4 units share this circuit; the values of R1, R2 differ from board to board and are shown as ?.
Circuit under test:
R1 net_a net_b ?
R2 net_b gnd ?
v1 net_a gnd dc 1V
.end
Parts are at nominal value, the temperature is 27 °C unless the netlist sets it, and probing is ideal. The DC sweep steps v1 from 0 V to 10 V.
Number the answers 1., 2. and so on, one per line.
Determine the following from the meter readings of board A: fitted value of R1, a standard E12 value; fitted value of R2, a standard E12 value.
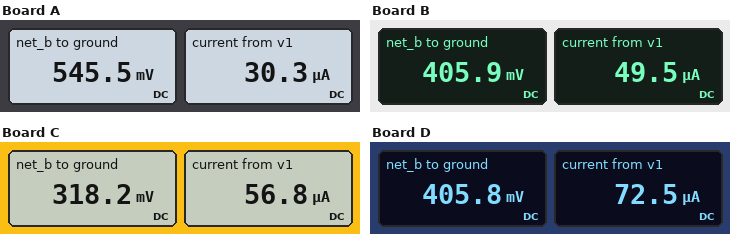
1. 15 kΩ
2. 18 kΩ
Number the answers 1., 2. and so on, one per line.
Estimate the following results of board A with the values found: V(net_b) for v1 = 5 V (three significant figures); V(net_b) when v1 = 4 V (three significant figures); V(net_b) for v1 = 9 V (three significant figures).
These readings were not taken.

1. 2.73 V
2. 2.18 V
3. 4.91 V
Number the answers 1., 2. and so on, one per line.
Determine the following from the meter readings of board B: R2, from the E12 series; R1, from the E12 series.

1. 8.2 kΩ
2. 12 kΩ
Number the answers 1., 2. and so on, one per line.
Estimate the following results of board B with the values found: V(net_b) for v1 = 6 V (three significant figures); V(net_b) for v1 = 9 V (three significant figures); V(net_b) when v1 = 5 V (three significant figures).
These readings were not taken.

1. 2.44 V
2. 3.65 V
3. 2.03 V
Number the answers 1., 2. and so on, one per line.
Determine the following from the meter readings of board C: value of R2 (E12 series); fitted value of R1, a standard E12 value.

1. 5.6 kΩ
2. 12 kΩ
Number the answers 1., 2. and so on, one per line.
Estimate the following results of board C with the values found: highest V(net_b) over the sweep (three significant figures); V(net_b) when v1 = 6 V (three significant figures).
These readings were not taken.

1. 3.18 V
2. 1.91 V
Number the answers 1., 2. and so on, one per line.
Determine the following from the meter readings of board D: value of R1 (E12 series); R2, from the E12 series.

1. 8.2 kΩ
2. 5.6 kΩ
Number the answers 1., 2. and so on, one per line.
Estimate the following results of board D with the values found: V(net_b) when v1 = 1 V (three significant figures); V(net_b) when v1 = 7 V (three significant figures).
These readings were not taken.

1. 406 mV
2. 2.84 V
